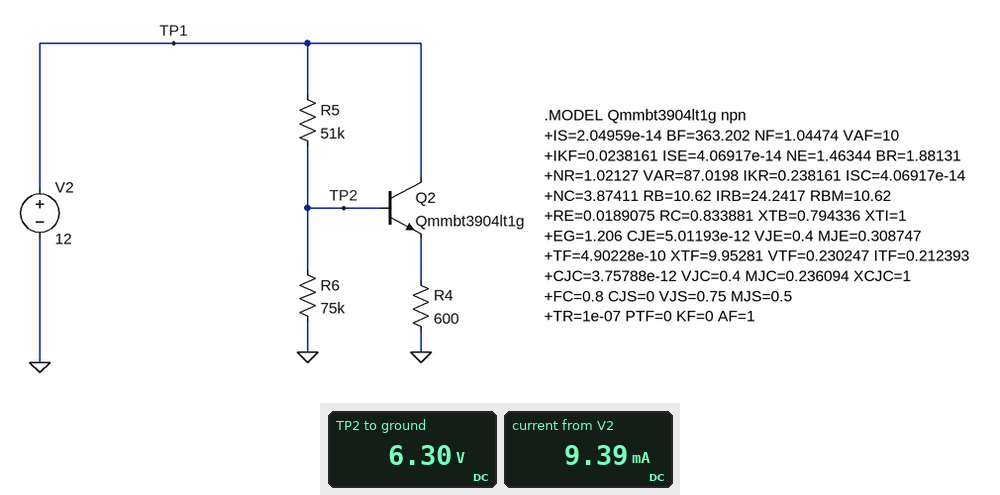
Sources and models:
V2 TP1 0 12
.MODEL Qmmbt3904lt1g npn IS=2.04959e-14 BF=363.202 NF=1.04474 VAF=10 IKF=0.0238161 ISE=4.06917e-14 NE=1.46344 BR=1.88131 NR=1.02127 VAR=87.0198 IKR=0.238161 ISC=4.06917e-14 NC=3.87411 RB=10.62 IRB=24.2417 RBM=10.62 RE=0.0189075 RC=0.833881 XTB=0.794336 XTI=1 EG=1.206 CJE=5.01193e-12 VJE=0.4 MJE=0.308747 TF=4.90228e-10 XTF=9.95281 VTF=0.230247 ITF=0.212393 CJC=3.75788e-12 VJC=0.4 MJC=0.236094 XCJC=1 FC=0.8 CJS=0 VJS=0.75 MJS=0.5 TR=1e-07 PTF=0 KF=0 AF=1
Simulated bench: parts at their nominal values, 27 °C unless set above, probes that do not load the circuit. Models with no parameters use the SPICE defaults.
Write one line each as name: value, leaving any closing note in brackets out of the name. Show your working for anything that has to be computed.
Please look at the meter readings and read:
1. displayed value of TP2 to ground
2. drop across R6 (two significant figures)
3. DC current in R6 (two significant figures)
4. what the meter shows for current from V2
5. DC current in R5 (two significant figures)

displayed value of TP2 to ground: 6.30 V
drop across R6: 6.3 V = 6.3 V
DC current in R6: (6.3 V) / 75 kΩ = 84 µA
what the meter shows for current from V2: 9.39 mA
DC current in R5: (12 V - 6.3 V) / 51 kΩ = 110 µA
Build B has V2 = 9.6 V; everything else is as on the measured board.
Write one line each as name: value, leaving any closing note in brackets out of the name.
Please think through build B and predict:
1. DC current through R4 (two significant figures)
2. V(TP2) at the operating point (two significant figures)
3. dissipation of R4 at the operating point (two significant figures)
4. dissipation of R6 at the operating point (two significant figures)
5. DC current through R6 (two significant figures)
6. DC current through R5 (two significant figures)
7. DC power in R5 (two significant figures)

DC current through R4: 7.2 mA
V(TP2) at the operating point: 5.0 V
dissipation of R4 at the operating point: 31 mW
dissipation of R6 at the operating point: 340 µW
DC current through R6: 67 µA
DC current through R5: 90 µA
DC power in R5: 410 µW
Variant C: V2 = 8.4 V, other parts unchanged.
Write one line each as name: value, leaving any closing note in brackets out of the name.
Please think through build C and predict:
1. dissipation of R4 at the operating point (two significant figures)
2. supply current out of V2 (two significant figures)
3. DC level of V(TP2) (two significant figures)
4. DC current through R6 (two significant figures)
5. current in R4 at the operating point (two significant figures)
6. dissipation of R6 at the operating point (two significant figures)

dissipation of R4 at the operating point: 23 mW
supply current out of V2: 6.2 mA
DC level of V(TP2): 4.4 V
DC current through R6: 59 µA
current in R4 at the operating point: 6.1 mA
dissipation of R6 at the operating point: 260 µW
